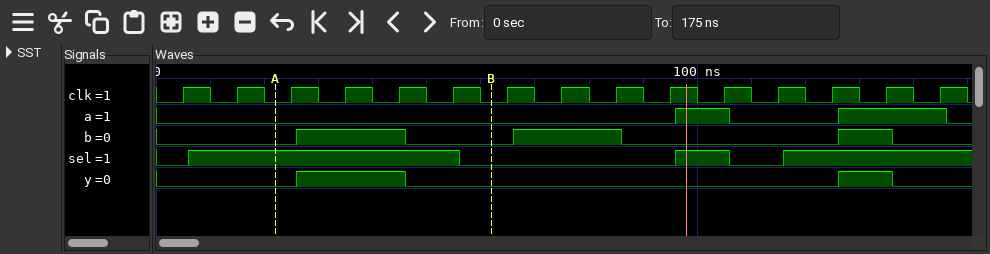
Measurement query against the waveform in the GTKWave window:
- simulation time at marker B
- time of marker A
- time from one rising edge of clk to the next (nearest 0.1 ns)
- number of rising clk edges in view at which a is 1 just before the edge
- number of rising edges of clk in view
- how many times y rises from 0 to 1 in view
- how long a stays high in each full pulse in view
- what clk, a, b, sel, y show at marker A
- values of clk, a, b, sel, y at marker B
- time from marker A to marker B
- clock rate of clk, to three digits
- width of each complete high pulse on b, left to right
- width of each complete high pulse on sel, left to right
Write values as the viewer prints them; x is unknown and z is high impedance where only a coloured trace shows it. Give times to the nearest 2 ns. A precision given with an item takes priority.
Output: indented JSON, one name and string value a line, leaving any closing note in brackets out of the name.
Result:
{
  "simulation time at marker B": "62 ns",
  "time of marker A": "22 ns",
  "time from one rising edge of clk to the next": "10 ns",
  "number of rising clk edges in view at which a is 1 just before the edge": "3",
  "number of rising edges of clk in view": "15",
  "how many times y rises from 0 to 1 in view": "2",
  "how long a stays high in each full pulse in view": "10 ns, 20 ns",
  "what clk, a, b, sel, y show at marker A": "clk=0, a=0, b=0, sel=1, y=0",
  "values of clk, a, b, sel, y at marker B": "clk=0, a=0, b=0, sel=0, y=0",
  "time from marker A to marker B": "40 ns",
  "clock rate of clk, to three digits": "100 MHz",
  "width of each complete high pulse on b, left to right": "20 ns, 20 ns, 10 ns",
  "width of each complete high pulse on sel, left to right": "50 ns, 10 ns"
}
